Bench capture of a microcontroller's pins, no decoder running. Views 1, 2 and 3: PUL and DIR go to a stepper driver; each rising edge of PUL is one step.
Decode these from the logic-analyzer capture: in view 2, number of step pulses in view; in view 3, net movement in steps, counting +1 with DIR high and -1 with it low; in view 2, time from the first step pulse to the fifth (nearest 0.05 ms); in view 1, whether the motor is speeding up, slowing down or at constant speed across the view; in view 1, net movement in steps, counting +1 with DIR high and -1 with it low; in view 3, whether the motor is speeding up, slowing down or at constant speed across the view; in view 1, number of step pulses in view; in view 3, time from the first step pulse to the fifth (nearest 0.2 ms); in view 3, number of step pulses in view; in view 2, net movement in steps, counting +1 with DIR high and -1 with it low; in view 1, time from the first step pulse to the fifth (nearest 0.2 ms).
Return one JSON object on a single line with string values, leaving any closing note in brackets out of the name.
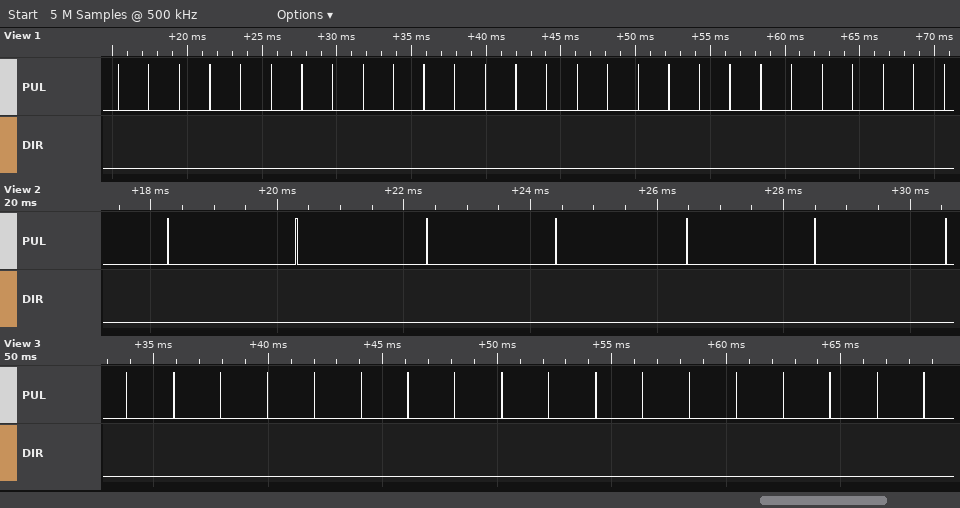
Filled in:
{"in view 2, number of step pulses in view": "7", "in view 3, net movement in steps, counting +1 with DIR high and -1 with it low": "-18", "in view 2, time from the first step pulse to the fifth": "8.20 ms", "in view 1, whether the motor is speeding up, slowing down or at constant speed across the view": "constant speed", "in view 1, net movement in steps, counting +1 with DIR high and -1 with it low": "-28", "in view 3, whether the motor is speeding up, slowing down or at constant speed across the view": "constant speed", "in view 1, number of step pulses in view": "28", "in view 3, time from the first step pulse to the fifth": "8.2 ms", "in view 3, number of step pulses in view": "18", "in view 2, net movement in steps, counting +1 with DIR high and -1 with it low": "-7", "in view 1, time from the first step pulse to the fifth": "8.2 ms"}
